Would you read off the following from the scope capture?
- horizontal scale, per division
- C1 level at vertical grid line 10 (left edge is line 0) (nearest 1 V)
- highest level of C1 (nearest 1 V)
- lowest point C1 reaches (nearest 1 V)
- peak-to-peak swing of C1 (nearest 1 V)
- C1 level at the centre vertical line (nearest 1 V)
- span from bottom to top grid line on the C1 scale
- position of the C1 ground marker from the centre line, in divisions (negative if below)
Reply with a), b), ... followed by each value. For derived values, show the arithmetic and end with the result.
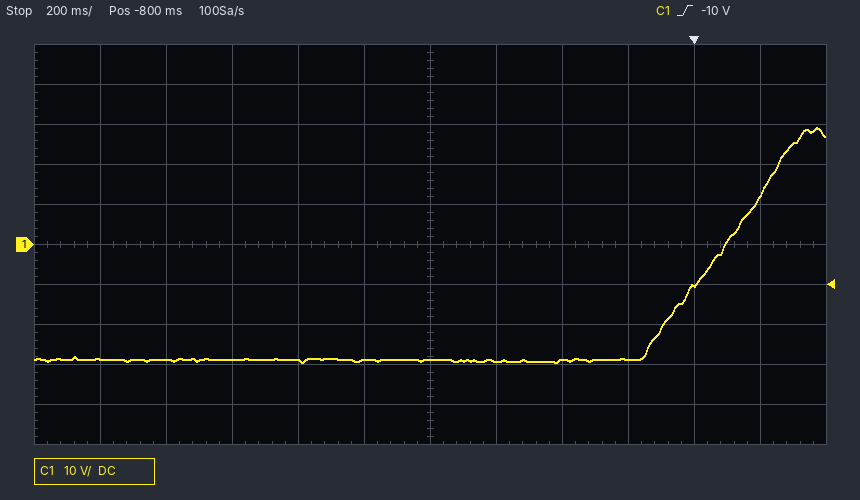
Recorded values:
a) 200 ms
b) -10 V
c) 29 V
d) -30 V
e) 29 V − (-30 V) = 59 V
f) -29 V
g) 100 V
h) 0.0 div
